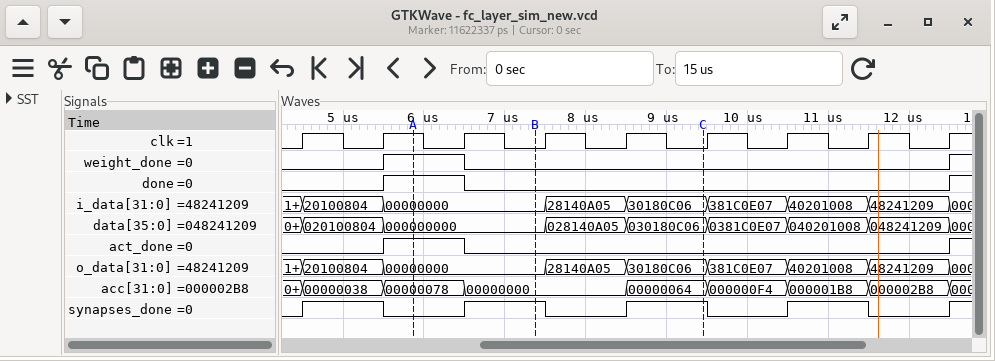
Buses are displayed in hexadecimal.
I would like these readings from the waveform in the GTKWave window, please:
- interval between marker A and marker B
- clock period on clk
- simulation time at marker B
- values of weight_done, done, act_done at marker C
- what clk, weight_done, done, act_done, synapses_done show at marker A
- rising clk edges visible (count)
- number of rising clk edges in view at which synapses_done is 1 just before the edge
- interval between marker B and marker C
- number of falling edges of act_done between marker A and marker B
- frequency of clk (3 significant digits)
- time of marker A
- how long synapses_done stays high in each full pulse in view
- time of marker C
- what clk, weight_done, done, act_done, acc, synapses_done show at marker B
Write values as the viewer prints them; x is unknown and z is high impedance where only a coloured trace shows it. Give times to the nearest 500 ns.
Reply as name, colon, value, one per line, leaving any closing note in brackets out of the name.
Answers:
interval between marker A and marker B: 1500 ns
clock period on clk: 1000 ns
simulation time at marker B: 7500 ns
values of weight_done, done, act_done at marker C: weight_done=0, done=0, act_done=0
what clk, weight_done, done, act_done, synapses_done show at marker A: clk=1, weight_done=1, done=1, act_done=1, synapses_done=0
rising clk edges visible: 9
number of rising clk edges in view at which synapses_done is 1 just before the edge: 4
interval between marker B and marker C: 2000 ns
number of falling edges of act_done between marker A and marker B: 1
frequency of clk: 1.00 MHz
time of marker A: 6000 ns
how long synapses_done stays high in each full pulse in view: 1000 ns, 1000 ns, 1000 ns, 1000 ns
time of marker C: 9500 ns
what clk, weight_done, done, act_done, acc, synapses_done show at marker B: clk=0, weight_done=0, done=0, act_done=0, acc=00000000, synapses_done=1
